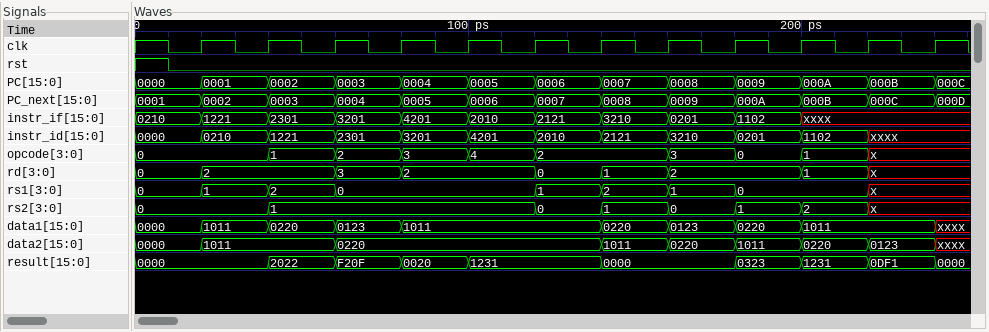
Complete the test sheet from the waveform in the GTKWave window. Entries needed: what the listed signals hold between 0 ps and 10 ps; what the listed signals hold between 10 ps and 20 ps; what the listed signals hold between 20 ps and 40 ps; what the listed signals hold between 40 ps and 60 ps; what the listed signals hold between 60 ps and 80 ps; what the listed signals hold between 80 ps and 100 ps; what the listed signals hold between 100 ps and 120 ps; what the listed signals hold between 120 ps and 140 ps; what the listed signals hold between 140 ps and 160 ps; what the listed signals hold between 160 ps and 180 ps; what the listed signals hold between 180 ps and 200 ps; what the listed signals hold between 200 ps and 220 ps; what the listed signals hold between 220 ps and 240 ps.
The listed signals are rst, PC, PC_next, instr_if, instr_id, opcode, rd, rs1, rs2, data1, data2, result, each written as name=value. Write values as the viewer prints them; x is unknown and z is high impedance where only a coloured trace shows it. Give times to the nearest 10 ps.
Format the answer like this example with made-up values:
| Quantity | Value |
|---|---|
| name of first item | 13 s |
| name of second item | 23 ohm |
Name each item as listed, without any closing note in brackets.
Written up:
| Quantity | Value |
|---|---|
| what the listed signals hold between 0 ps and 10 ps | rst=1, PC=0000, PC_next=0001, instr_if=0210, instr_id=0000, opcode=0, rd=0, rs1=0, rs2=0, data1=0000, data2=0000, result=0000 |
| what the listed signals hold between 10 ps and 20 ps | rst=0, PC=0000, PC_next=0001, instr_if=0210, instr_id=0000, opcode=0, rd=0, rs1=0, rs2=0, data1=0000, data2=0000, result=0000 |
| what the listed signals hold between 20 ps and 40 ps | rst=0, PC=0001, PC_next=0002, instr_if=1221, instr_id=0210, opcode=0, rd=2, rs1=1, rs2=0, data1=1011, data2=1011, result=0000 |
| what the listed signals hold between 40 ps and 60 ps | rst=0, PC=0002, PC_next=0003, instr_if=2301, instr_id=1221, opcode=1, rd=2, rs1=2, rs2=1, data1=0220, data2=1011, result=2022 |
| what the listed signals hold between 60 ps and 80 ps | rst=0, PC=0003, PC_next=0004, instr_if=3201, instr_id=2301, opcode=2, rd=3, rs1=0, rs2=1, data1=0123, data2=0220, result=F20F |
| what the listed signals hold between 80 ps and 100 ps | rst=0, PC=0004, PC_next=0005, instr_if=4201, instr_id=3201, opcode=3, rd=2, rs1=0, rs2=1, data1=1011, data2=0220, result=0020 |
| what the listed signals hold between 100 ps and 120 ps | rst=0, PC=0005, PC_next=0006, instr_if=2010, instr_id=4201, opcode=4, rd=2, rs1=0, rs2=1, data1=1011, data2=0220, result=1231 |
| what the listed signals hold between 120 ps and 140 ps | rst=0, PC=0006, PC_next=0007, instr_if=2121, instr_id=2010, opcode=2, rd=0, rs1=1, rs2=0, data1=1011, data2=0220, result=1231 |
| what the listed signals hold between 140 ps and 160 ps | rst=0, PC=0007, PC_next=0008, instr_if=3210, instr_id=2121, opcode=2, rd=1, rs1=2, rs2=1, data1=0220, data2=1011, result=0000 |
| what the listed signals hold between 160 ps and 180 ps | rst=0, PC=0008, PC_next=0009, instr_if=0201, instr_id=3210, opcode=3, rd=2, rs1=1, rs2=0, data1=0123, data2=0220, result=0000 |
| what the listed signals hold between 180 ps and 200 ps | rst=0, PC=0009, PC_next=000A, instr_if=1102, instr_id=0201, opcode=0, rd=2, rs1=0, rs2=1, data1=0220, data2=1011, result=0323 |
| what the listed signals hold between 200 ps and 220 ps | rst=0, PC=000A, PC_next=000B, instr_if=xxxx, instr_id=1102, opcode=1, rd=1, rs1=0, rs2=2, data1=1011, data2=0220, result=1231 |
| what the listed signals hold between 220 ps and 240 ps | rst=0, PC=000B, PC_next=000C, instr_if=xxxx, instr_id=xxxx, opcode=x, rd=x, rs1=x, rs2=x, data1=1011, data2=0123, result=0DF1 |
